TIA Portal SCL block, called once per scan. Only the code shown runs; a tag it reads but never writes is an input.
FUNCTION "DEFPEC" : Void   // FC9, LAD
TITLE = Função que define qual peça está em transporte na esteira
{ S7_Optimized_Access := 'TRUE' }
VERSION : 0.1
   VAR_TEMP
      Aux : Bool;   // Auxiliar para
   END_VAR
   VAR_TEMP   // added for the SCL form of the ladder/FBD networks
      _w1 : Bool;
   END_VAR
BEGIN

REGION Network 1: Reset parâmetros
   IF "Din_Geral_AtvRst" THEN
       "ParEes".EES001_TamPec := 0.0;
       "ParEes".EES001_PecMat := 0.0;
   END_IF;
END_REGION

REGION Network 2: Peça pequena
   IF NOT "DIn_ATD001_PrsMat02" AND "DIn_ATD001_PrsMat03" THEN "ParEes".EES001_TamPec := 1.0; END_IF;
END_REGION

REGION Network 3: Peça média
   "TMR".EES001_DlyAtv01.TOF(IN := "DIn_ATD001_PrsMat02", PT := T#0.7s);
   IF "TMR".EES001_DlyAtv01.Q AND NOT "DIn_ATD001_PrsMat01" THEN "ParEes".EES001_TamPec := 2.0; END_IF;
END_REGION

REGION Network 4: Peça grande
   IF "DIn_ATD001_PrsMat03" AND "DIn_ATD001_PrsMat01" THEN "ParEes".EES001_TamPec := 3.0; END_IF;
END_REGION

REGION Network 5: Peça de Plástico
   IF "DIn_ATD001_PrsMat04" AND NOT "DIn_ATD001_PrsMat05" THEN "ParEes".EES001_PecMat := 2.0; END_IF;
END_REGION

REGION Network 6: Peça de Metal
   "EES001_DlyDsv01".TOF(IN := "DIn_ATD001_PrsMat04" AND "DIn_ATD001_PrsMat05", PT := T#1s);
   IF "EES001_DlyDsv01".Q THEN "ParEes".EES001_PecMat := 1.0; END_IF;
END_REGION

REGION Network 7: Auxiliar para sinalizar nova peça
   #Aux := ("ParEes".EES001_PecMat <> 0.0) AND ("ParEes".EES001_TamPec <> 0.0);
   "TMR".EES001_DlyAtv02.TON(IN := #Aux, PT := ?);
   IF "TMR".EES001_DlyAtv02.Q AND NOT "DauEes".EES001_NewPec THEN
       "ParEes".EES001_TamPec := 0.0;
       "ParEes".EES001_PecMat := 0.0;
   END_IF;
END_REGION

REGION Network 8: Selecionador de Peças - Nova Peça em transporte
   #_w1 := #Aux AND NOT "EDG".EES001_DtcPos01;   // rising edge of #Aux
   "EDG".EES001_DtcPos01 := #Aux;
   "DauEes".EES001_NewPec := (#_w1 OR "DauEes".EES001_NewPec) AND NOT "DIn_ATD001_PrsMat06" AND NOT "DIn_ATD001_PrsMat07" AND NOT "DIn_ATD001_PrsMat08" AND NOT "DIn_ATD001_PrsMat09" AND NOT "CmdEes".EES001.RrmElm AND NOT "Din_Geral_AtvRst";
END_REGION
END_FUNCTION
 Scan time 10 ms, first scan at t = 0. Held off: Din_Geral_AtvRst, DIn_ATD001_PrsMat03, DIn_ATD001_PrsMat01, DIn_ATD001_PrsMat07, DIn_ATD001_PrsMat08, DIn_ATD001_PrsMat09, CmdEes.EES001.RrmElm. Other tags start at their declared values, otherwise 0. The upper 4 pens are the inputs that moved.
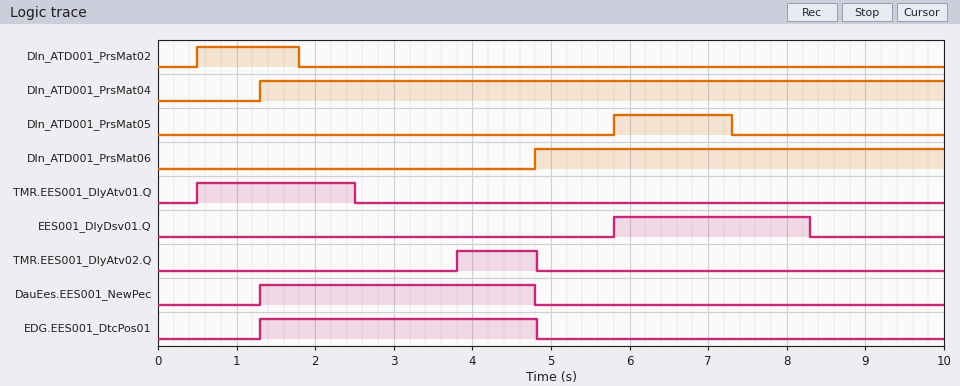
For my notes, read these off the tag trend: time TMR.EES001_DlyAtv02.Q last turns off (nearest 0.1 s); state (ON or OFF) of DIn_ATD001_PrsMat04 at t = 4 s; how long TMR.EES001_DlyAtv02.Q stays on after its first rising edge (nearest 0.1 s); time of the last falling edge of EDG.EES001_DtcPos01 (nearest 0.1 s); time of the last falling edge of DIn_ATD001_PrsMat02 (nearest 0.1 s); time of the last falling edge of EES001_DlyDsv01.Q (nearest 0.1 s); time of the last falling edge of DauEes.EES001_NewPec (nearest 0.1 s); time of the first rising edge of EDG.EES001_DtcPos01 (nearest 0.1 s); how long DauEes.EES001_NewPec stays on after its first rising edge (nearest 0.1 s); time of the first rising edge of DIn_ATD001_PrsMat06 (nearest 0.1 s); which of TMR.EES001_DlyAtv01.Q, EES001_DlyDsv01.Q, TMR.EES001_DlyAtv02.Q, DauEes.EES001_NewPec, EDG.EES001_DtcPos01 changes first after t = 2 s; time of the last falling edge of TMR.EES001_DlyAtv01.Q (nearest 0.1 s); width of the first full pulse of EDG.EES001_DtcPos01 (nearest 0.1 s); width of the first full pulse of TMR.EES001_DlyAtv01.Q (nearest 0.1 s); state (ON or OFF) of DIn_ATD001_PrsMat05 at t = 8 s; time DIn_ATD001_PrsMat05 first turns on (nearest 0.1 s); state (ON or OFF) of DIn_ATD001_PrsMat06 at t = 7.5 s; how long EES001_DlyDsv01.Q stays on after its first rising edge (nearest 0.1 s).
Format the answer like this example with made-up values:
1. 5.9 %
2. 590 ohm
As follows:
1. 4.8 s
2. ON
3. 1.0 s
4. 4.8 s
5. 1.8 s
6. 8.3 s
7. 4.8 s
8. 1.3 s
9. 3.5 s
10. 4.8 s
11. TMR.EES001_DlyAtv01.Q
12. 2.5 s
13. 3.5 s
14. 2.0 s
15. OFF
16. 5.8 s
17. ON
18. 2.5 s
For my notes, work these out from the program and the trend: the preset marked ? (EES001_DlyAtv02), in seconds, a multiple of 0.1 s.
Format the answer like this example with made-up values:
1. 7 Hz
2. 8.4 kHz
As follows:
1. 2.5 s
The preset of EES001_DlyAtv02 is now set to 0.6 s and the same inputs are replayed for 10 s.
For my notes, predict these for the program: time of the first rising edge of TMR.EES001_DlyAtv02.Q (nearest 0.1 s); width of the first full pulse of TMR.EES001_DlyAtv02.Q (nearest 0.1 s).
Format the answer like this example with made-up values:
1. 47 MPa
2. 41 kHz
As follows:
1. 1.9 s
2. 2.9 s
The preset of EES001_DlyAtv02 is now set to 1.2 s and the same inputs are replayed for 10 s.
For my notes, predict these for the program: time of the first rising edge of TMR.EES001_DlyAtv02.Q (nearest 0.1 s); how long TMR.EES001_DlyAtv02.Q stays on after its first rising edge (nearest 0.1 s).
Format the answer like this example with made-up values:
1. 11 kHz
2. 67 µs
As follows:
1. 2.5 s
2. 2.3 s
